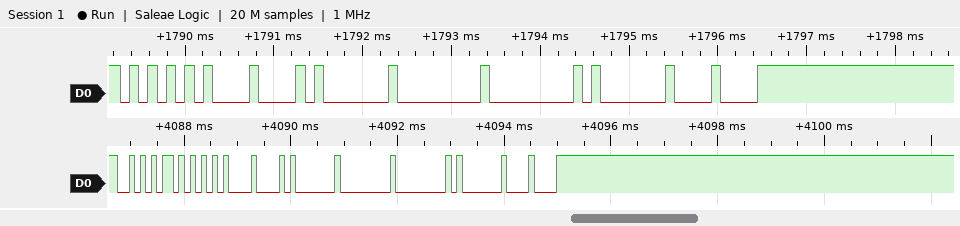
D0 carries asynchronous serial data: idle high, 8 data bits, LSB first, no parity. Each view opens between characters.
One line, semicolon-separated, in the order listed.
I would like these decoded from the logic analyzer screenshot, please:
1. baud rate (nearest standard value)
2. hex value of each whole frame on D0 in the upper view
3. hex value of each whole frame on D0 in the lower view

9600 baud; 55, 08, 01, 00, 00, 01, 08; AA, 55, 08, 01, 00, 00, 01, 08
